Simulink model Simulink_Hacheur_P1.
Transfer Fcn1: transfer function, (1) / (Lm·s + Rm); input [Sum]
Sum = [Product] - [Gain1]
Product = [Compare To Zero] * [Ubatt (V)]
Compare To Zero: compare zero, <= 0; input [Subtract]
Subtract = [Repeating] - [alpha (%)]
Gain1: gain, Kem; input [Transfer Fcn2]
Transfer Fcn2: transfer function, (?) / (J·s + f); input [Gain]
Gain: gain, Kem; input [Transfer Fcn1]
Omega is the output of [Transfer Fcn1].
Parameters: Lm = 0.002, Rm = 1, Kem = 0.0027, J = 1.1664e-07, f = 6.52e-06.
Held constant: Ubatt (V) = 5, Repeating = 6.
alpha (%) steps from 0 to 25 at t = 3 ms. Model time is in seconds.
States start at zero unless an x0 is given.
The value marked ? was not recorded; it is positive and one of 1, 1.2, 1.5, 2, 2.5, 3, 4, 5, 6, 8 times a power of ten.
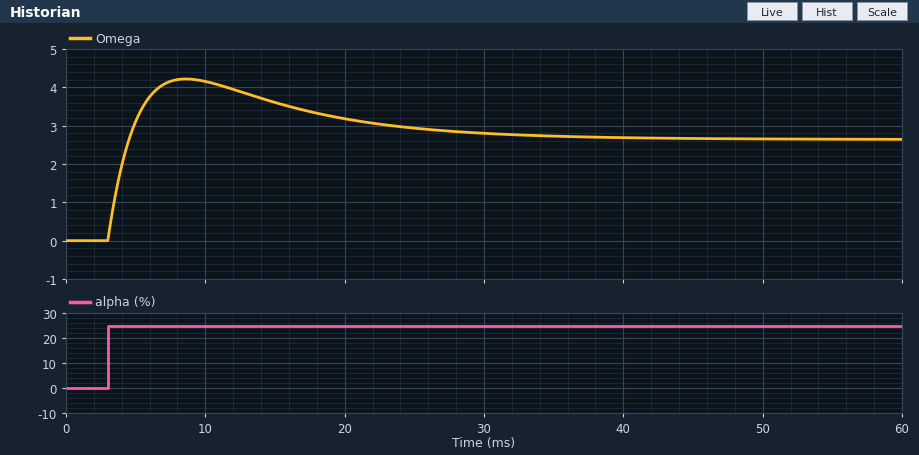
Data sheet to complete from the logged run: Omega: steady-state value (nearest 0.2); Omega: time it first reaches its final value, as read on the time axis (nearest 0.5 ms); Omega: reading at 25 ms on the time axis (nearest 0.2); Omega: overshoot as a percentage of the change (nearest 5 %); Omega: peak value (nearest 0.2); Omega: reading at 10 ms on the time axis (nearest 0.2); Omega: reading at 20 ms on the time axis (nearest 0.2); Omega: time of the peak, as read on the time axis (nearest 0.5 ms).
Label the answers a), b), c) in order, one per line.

a) 2.6
b) 4.5 ms
c) 3.0
d) 60 %
e) 4.2
f) 4.2
g) 3.2
h) 8.5 ms
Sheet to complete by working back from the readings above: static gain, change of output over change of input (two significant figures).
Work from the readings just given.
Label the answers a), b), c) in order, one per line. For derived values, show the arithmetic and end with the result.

a) (2.6 - 0) / (25 - 0) = 0.10
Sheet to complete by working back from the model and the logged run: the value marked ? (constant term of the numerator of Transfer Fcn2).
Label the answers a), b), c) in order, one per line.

a) 0.8
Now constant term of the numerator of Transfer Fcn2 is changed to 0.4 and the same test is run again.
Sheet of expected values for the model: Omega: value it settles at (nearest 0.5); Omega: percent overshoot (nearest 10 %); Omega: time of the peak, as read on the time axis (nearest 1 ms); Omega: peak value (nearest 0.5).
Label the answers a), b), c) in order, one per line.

a) 3.5
b) 30 %
c) 10 ms
d) 4.5
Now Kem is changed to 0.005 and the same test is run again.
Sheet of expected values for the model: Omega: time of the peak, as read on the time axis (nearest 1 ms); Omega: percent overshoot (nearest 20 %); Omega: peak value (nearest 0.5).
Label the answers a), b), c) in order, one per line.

a) 7 ms
b) 180 %
c) 3.5
